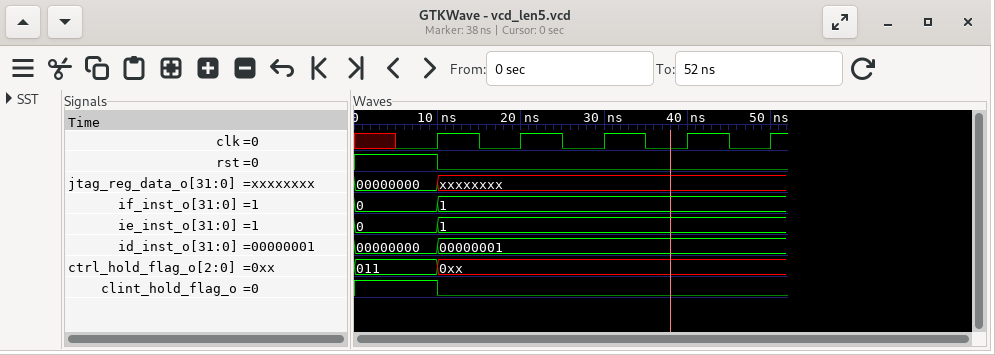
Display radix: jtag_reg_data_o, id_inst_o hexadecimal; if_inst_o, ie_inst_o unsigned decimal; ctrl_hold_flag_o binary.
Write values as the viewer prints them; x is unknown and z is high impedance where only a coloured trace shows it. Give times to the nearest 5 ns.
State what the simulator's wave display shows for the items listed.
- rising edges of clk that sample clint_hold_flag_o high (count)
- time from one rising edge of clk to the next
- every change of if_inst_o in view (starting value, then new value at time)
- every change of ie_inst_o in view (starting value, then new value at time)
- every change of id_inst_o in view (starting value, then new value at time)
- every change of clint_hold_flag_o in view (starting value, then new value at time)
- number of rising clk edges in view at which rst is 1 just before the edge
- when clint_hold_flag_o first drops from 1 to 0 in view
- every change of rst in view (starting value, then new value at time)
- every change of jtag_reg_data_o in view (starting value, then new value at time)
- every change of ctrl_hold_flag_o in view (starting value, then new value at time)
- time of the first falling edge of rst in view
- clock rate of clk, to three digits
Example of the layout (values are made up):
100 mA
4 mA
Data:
1
10 ns
0, 1 at 10 ns
0, 1 at 10 ns
00000000, 00000001 at 10 ns
1, 0 at 10 ns
1
10 ns
1, 0 at 10 ns
00000000, xxxxxxxx at 10 ns
011, 0xx at 10 ns
10 ns
100 MHz
